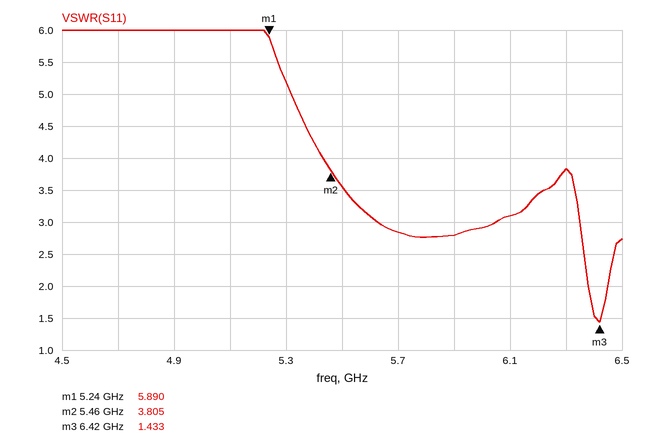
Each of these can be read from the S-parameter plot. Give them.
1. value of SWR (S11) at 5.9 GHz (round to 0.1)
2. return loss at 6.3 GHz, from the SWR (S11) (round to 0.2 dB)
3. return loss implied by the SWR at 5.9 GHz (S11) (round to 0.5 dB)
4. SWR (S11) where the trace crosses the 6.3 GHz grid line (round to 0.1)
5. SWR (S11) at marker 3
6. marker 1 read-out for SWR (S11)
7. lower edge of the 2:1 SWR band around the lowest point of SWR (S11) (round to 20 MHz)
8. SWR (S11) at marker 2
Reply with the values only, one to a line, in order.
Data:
2.8
4.6 dB
6.5 dB
3.8
1.433
5.890
6.38 GHz
3.805
